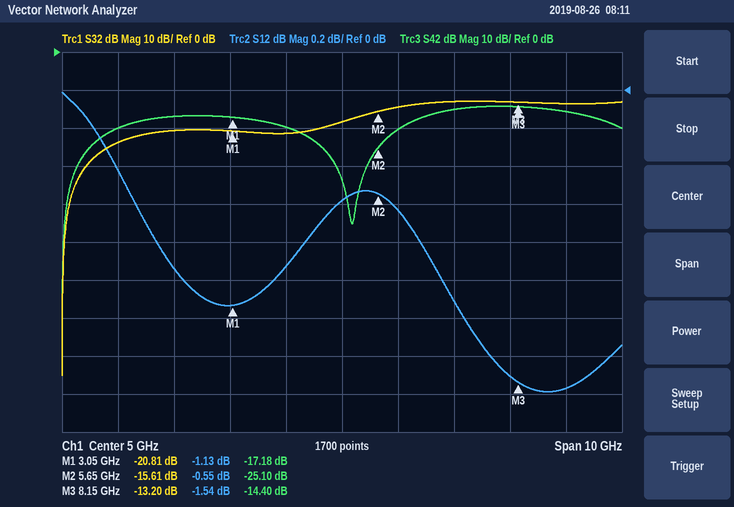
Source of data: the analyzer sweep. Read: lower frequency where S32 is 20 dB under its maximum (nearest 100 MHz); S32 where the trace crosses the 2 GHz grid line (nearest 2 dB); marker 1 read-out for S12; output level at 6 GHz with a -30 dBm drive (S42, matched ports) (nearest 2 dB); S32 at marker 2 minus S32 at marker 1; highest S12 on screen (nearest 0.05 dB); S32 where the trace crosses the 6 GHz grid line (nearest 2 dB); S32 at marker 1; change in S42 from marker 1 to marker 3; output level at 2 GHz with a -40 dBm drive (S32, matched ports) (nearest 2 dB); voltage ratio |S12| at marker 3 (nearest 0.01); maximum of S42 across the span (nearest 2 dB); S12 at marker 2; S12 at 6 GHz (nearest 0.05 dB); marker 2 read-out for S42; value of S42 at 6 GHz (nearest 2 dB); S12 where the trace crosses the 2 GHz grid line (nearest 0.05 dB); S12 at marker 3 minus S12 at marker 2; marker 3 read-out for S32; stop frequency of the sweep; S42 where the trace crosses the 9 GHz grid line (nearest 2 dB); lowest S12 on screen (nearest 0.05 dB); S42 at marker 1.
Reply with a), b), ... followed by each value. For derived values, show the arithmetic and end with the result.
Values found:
a) 300 MHz
b) -20 dB
c) -1.13 dB
d) -30 dBm + (-20 dB) = -50 dBm
e) -15.61 − (-20.81) = 5.20 dB
f) 0.00 dB
g) -14 dB
h) -20.81 dB
i) -14.4 − (-17.18) = 2.78 dB
j) -40 dBm + (-20 dB) = -60 dBm
k) 10^(-1.54/20) ≈ 0.84
l) -14 dB
m) -0.55 dB
n) -0.65 dB
o) -25.10 dB
p) -20 dB
q) -0.95 dB
r) -1.54 − (-0.55) = -0.99 dB
s) -13.20 dB
t) 10 GHz
u) -16 dB
v) -1.60 dB
w) -17.18 dB
